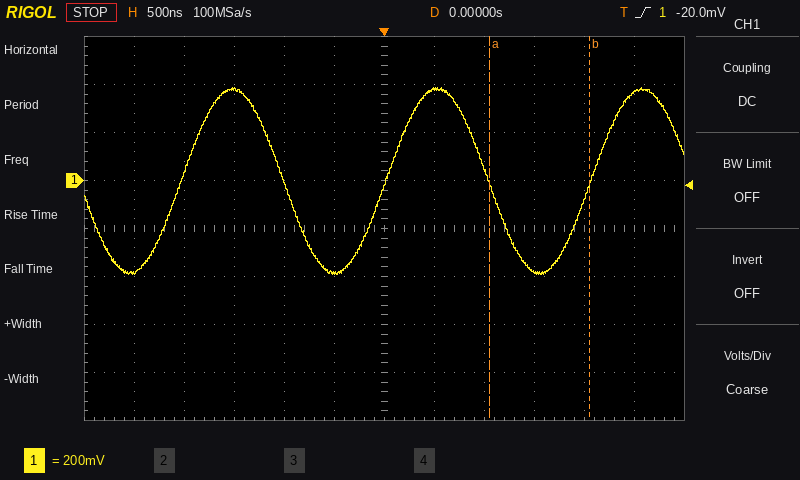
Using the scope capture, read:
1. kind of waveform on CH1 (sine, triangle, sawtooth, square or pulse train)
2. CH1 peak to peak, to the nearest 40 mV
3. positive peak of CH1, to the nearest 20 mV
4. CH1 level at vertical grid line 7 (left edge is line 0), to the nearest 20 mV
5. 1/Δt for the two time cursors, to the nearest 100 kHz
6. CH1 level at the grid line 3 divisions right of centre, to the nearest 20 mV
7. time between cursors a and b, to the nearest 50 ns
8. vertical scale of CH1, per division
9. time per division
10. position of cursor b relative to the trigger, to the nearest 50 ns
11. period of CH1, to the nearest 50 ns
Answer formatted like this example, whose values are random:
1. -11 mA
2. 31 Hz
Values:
1. sine
2. 760 mV
3. 380 mV
4. 380 mV
5. 1.0 MHz
6. -380 mV
7. 1.00 µs
8. 200 mV
9. 500 ns
10. +2.05 µs
11. 2.05 µs
